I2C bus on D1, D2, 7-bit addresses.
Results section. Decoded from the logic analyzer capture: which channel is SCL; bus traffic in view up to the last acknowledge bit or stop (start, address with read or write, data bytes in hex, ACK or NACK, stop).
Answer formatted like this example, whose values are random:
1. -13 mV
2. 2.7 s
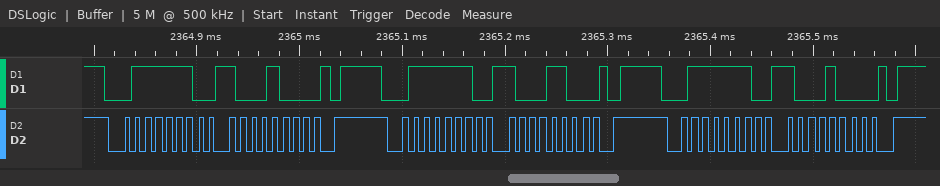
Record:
1. D2
2. start, address 3F write ACK, 88 ACK, stop, start, address 3F write ACK, 8C ACK, stop, start, address 3F write ACK, 88 ACK, stop
